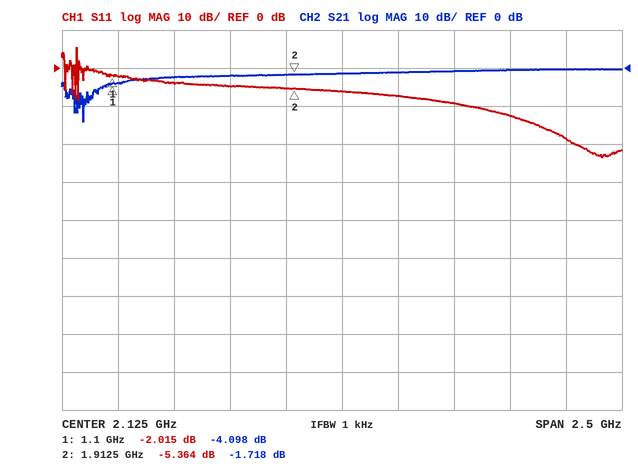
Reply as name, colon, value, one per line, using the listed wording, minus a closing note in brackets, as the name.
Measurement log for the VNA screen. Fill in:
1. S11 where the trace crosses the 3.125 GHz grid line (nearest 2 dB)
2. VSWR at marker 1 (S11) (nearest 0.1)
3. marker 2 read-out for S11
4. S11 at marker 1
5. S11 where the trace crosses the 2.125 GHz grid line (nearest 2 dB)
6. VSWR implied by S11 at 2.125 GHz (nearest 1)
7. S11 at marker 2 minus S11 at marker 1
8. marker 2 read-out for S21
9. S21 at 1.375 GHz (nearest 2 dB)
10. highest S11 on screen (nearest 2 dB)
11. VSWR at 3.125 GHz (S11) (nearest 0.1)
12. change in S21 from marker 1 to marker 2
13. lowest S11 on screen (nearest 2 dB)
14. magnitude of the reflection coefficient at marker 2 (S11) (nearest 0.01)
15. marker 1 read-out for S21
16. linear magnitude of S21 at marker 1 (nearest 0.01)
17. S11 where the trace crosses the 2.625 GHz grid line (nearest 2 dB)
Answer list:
S11 where the trace crosses the 3.125 GHz grid line: -18 dB
VSWR at marker 1 (S11): 8.7
marker 2 read-out for S11: -5.364 dB
S11 at marker 1: -2.015 dB
S11 where the trace crosses the 2.125 GHz grid line: -6 dB
VSWR implied by S11 at 2.125 GHz: 3
S11 at marker 2 minus S11 at marker 1: -3.349 dB
marker 2 read-out for S21: -1.718 dB
S21 at 1.375 GHz: -2 dB
highest S11 on screen: 6 dB
VSWR at 3.125 GHz (S11): 1.3
change in S21 from marker 1 to marker 2: 2.380 dB
lowest S11 on screen: -24 dB
magnitude of the reflection coefficient at marker 2 (S11): 0.54
marker 1 read-out for S21: -4.098 dB
linear magnitude of S21 at marker 1: 0.62
S11 where the trace crosses the 2.625 GHz grid line: -10 dB
